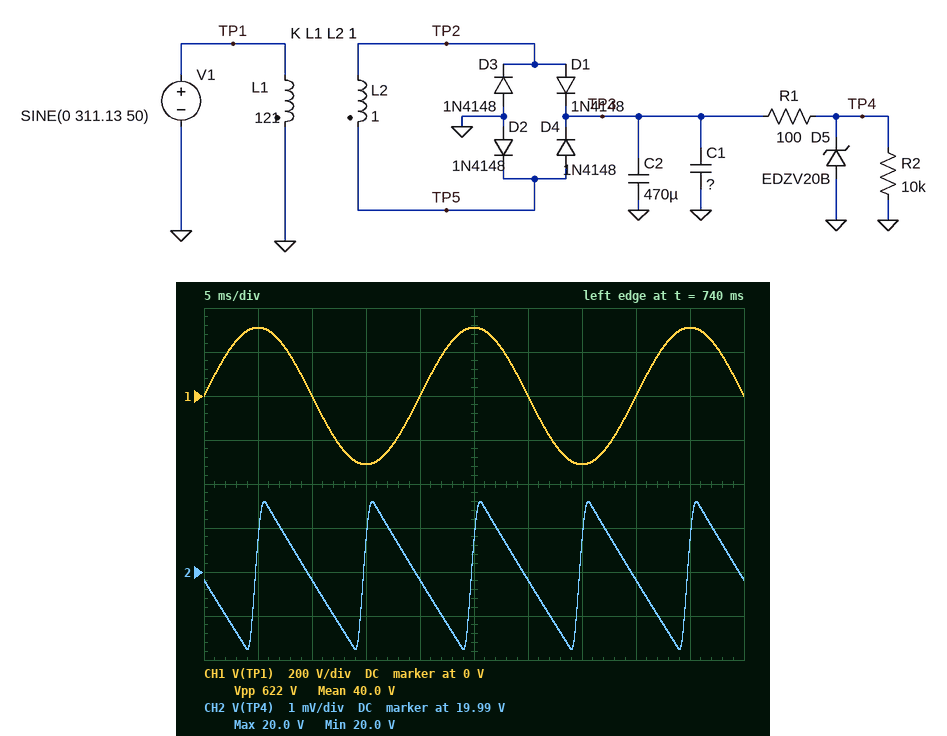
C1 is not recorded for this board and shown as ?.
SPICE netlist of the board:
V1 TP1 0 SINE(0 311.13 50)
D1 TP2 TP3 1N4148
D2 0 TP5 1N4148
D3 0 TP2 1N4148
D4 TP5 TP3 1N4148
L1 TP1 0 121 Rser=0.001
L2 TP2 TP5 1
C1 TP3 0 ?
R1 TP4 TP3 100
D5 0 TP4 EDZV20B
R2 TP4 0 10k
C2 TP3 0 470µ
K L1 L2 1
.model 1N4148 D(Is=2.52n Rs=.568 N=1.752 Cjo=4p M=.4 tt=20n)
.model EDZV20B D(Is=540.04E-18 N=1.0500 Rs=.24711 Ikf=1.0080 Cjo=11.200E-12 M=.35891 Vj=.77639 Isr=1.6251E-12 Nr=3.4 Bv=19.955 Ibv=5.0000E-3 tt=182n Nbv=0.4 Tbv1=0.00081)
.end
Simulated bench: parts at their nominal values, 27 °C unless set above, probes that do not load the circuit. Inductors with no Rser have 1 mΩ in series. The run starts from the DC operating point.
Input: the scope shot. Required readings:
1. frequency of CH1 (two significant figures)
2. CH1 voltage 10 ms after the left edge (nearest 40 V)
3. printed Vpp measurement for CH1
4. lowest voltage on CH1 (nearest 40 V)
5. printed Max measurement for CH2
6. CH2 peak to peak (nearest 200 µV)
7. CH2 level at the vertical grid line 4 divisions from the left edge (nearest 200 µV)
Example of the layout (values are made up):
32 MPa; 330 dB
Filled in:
50 Hz; 0 V; 622 V; -320 V; 20.0 V; 3.4 mV; 19.9938 V
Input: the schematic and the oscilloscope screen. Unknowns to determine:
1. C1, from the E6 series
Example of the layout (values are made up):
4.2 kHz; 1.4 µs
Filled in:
150 µF
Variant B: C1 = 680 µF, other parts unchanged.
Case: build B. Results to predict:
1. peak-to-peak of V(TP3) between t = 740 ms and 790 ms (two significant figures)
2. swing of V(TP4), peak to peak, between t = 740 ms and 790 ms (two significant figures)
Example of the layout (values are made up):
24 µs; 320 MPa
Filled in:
430 mV; 1.8 mV
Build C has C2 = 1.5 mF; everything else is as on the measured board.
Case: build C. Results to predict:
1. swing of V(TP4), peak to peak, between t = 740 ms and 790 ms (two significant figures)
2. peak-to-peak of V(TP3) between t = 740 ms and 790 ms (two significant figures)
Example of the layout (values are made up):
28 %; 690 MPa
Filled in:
1.3 mV; 300 mV
